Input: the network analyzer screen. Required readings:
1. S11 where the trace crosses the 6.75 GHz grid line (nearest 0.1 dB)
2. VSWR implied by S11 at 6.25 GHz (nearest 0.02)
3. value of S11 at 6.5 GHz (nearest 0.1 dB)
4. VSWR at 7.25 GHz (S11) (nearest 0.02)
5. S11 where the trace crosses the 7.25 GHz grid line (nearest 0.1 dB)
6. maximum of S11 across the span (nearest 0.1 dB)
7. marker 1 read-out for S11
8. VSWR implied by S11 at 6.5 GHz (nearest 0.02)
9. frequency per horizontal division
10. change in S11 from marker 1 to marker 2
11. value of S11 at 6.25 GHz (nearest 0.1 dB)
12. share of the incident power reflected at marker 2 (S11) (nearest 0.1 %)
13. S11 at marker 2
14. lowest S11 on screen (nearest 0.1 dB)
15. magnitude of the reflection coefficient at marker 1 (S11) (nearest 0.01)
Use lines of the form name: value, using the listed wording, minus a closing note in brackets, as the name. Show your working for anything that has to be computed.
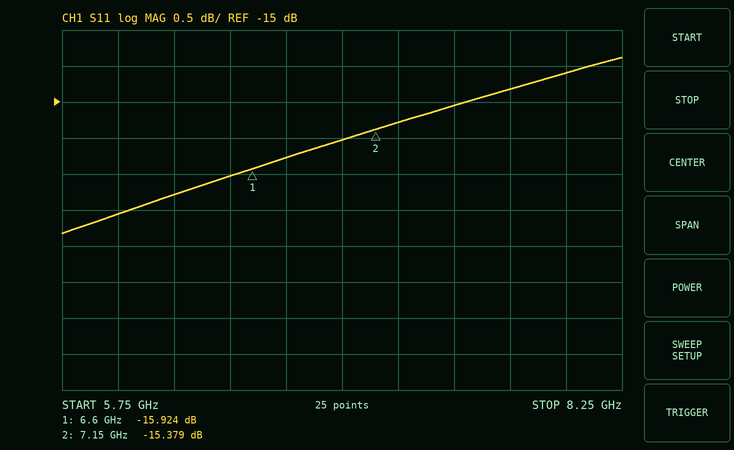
S11 where the trace crosses the 6.75 GHz grid line: -15.8 dB
VSWR implied by S11 at 6.25 GHz: |Γ| = 10^(-16.3/20) = 0.1531; VSWR = (1 + 0.1531)/(1 − 0.1531) ≈ 1.36
value of S11 at 6.5 GHz: -16.0 dB
VSWR at 7.25 GHz (S11): |Γ| = 10^(-15.3/20) = 0.1718; VSWR = (1 + 0.1718)/(1 − 0.1718) ≈ 1.41, so 1.42 to the nearest 0.02
S11 where the trace crosses the 7.25 GHz grid line: -15.3 dB
maximum of S11 across the span: -14.4 dB
marker 1 read-out for S11: -15.924 dB
VSWR implied by S11 at 6.5 GHz: |Γ| = 10^(-16/20) = 0.1585; VSWR = (1 + 0.1585)/(1 − 0.1585) ≈ 1.38
frequency per horizontal division: 250 MHz
change in S11 from marker 1 to marker 2: -15.379 − (-15.924) = 0.545 dB
value of S11 at 6.25 GHz: -16.3 dB
share of the incident power reflected at marker 2 (S11): 10^(-15.379/10) ≈ 2.9 %
S11 at marker 2: -15.379 dB
lowest S11 on screen: -16.8 dB
magnitude of the reflection coefficient at marker 1 (S11): 10^(-15.924/20) ≈ 0.16
